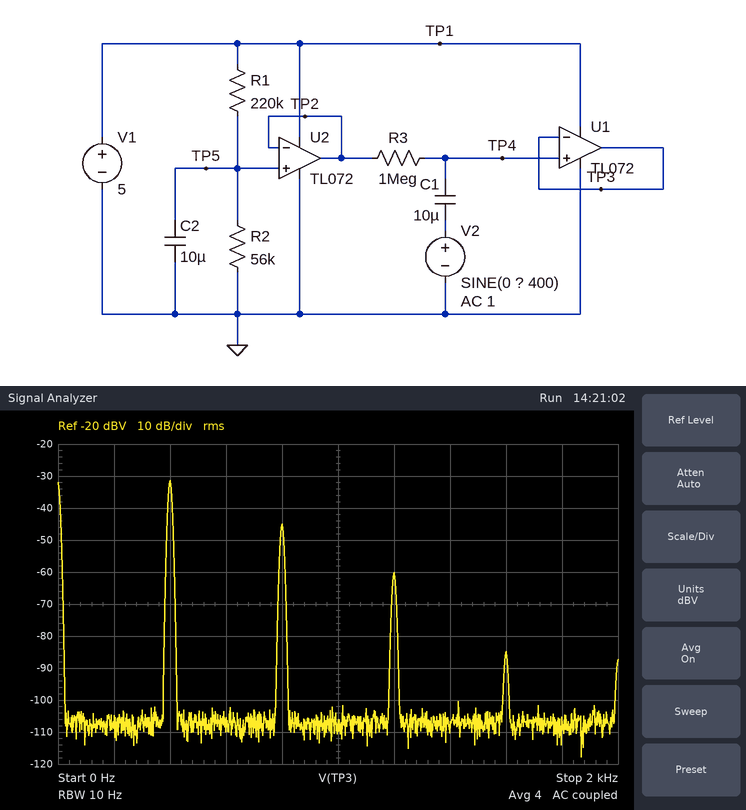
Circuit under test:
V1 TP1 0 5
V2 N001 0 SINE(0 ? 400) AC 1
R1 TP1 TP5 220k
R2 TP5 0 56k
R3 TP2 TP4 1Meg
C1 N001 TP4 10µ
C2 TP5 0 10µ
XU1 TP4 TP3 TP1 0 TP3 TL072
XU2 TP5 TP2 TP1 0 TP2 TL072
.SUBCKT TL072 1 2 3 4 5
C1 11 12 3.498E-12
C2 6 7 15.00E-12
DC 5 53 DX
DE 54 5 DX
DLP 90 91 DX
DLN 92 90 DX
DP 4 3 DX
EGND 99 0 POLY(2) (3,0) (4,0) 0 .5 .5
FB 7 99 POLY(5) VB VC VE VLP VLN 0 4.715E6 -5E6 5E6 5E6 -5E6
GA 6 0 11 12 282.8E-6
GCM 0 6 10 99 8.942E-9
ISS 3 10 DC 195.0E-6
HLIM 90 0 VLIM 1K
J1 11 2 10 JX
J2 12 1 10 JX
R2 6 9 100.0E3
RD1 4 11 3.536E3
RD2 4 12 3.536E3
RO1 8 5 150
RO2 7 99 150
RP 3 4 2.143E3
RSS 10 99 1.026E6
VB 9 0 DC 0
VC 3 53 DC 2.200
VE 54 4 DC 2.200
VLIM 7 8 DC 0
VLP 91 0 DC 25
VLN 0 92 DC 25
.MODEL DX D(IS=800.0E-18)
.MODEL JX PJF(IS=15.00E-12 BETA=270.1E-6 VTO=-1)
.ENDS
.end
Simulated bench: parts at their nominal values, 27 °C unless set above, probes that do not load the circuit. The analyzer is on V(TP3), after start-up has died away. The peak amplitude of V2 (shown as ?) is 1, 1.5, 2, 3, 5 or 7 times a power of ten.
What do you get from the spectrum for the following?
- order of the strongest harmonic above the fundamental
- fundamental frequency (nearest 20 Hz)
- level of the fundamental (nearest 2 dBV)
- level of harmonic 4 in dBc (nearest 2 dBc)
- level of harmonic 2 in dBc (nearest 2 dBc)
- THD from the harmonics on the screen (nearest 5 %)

2
400 Hz
-32 dBV
-54 dBc
-14 dBc
20 %
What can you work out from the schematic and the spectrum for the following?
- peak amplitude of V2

100 mV
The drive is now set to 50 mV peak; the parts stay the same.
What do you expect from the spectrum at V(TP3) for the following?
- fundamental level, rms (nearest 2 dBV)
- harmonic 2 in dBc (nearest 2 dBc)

-38 dBV
-20 dBc
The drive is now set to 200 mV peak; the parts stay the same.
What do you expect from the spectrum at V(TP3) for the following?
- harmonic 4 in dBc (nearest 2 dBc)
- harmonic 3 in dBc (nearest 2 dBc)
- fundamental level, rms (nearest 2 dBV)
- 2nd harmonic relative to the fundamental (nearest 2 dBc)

-36 dBc
-26 dBc
-24 dBV
-10 dBc
